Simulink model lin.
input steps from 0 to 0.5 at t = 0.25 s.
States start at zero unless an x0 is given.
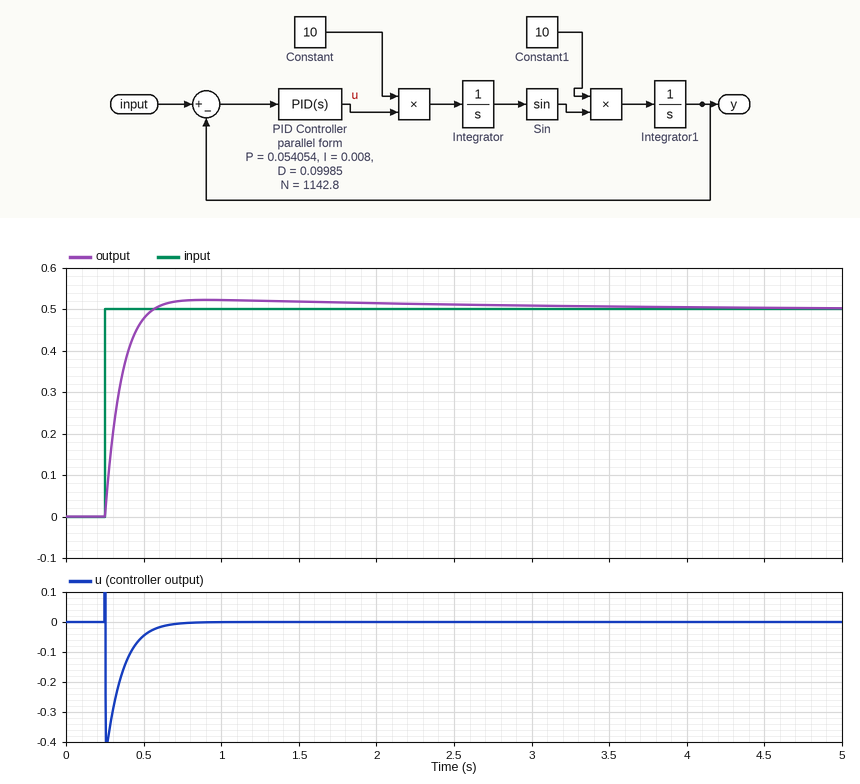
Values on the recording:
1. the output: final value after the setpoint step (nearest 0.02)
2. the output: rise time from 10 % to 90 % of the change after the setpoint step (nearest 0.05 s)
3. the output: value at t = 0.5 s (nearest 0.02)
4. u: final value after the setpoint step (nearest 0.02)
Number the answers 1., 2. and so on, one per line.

1. 0.50
2. 0.20 s
3. 0.48
4. 0.00
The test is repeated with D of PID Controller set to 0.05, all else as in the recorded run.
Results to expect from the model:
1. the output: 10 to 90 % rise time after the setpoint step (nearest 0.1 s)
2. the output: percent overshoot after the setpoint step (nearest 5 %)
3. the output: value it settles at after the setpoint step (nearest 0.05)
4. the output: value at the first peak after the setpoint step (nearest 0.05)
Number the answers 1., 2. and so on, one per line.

1. 0.3 s
2. 15 %
3. 0.50
4. 0.55
